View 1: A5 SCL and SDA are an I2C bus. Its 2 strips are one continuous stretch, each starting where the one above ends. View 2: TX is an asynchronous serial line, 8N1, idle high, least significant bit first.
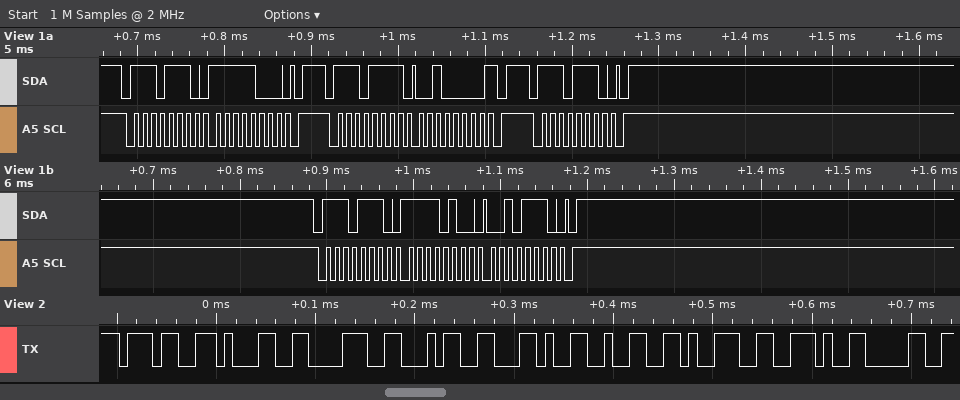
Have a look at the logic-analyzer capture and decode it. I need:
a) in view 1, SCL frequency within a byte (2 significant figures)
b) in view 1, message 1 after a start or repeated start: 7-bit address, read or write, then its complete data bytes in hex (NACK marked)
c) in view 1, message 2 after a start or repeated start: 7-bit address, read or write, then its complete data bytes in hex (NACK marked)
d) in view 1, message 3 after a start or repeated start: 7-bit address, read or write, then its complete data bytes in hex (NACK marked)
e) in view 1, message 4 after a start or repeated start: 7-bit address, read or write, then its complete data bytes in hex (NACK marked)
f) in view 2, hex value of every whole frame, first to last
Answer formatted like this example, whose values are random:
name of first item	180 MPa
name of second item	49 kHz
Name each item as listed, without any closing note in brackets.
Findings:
in view 1, SCL frequency within a byte	100 kHz
in view 1, message 1 after a start or repeated start: 7-bit address, read or write, then its complete data bytes in hex	0x77 write: F8
in view 1, message 2 after a start or repeated start: 7-bit address, read or write, then its complete data bytes in hex	0x77 read: 20 NACK
in view 1, message 3 after a start or repeated start: 7-bit address, read or write, then its complete data bytes in hex	0x77 write
in view 1, message 4 after a start or repeated start: 7-bit address, read or write, then its complete data bytes in hex	0x77 write: F4 2E
in view 2, hex value of every whole frame, first to last	37 31 38 34 2C 32 39 2E 30
